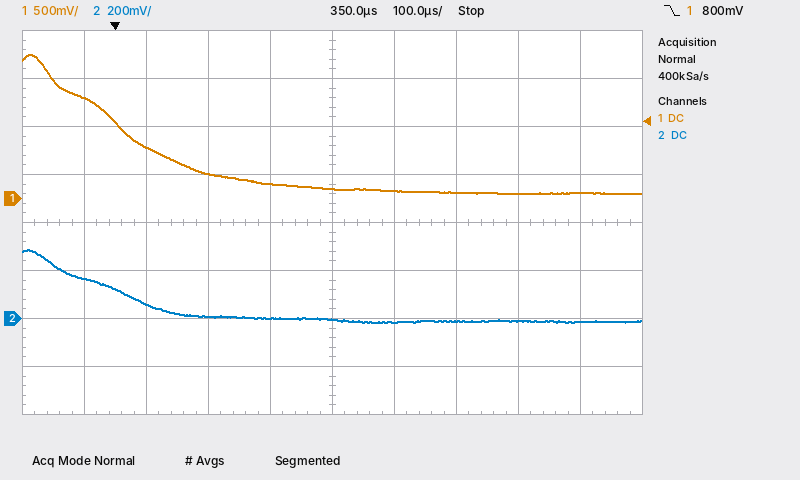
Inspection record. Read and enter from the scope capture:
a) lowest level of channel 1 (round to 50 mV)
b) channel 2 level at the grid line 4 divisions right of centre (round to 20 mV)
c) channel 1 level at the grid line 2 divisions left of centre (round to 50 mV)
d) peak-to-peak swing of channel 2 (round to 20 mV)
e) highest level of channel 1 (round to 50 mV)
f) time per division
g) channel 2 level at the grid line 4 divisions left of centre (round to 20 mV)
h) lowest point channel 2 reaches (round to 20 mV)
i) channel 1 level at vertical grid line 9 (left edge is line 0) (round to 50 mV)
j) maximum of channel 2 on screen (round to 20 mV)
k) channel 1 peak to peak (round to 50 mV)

50 mV
-20 mV
250 mV
300 mV
1.50 V
100 µs
160 mV
-20 mV
50 mV
280 mV
1.45 V
